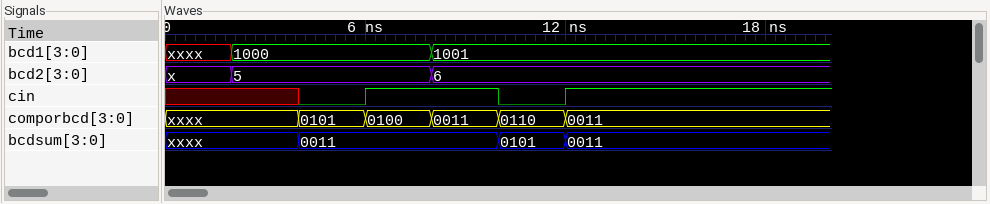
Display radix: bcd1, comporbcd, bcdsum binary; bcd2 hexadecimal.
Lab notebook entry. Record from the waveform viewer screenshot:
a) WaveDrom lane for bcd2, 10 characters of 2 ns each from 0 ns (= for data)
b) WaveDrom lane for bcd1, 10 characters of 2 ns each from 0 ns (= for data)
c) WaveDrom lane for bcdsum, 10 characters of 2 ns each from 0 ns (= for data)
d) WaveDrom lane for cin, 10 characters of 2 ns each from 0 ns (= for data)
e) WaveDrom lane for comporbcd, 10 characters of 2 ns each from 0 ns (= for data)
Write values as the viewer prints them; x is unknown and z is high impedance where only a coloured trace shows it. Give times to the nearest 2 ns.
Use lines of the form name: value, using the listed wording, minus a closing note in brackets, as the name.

WaveDrom lane for bcd2, 10 characters of 2 ns each from 0 ns: {name: 'bcd2', wave: 'x=..=.....', data: '5 6'}
WaveDrom lane for bcd1, 10 characters of 2 ns each from 0 ns: {name: 'bcd1', wave: 'x=..=.....', data: '1000 1001'}
WaveDrom lane for bcdsum, 10 characters of 2 ns each from 0 ns: {name: 'bcdsum', wave: 'x.=..==...', data: '0011 0101 0011'}
WaveDrom lane for cin, 10 characters of 2 ns each from 0 ns: {name: 'cin', wave: 'x.01.01...'}
WaveDrom lane for comporbcd, 10 characters of 2 ns each from 0 ns: {name: 'comporbcd', wave: 'x.=====...', data: '0101 0100 0011 0110 0011'}
